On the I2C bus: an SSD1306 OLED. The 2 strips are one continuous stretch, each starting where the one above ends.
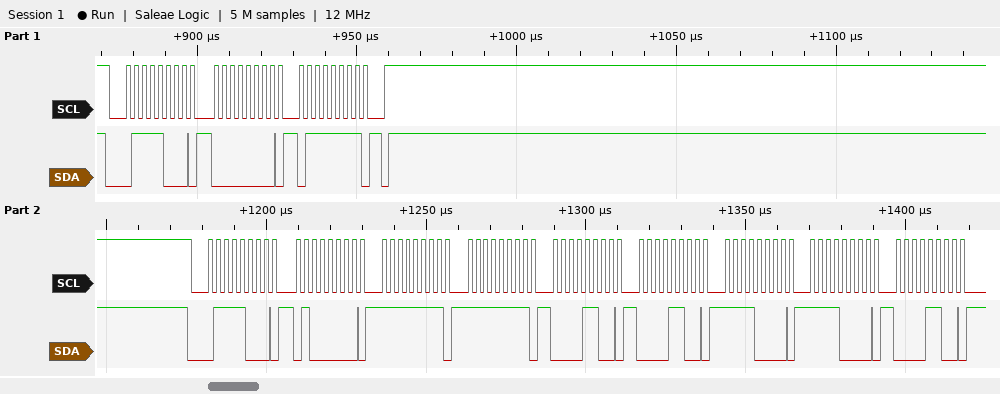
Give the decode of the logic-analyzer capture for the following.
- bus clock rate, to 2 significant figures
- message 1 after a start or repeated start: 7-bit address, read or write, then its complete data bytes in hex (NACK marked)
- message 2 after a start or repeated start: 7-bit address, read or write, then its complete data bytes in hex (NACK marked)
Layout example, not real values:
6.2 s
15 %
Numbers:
400 kHz
0x3C write: 00 7F
0x3C write: 40 FF FF 0C 0C F0 F0 0C
